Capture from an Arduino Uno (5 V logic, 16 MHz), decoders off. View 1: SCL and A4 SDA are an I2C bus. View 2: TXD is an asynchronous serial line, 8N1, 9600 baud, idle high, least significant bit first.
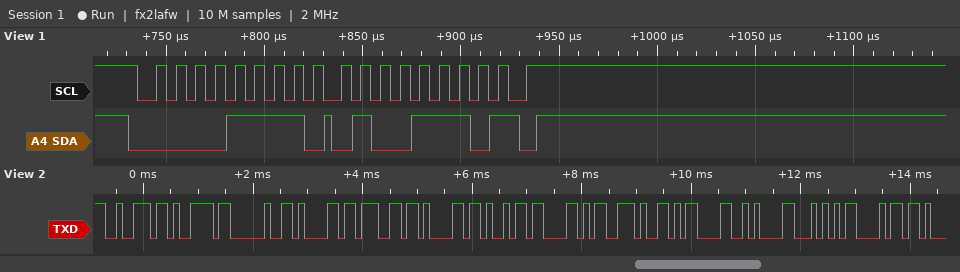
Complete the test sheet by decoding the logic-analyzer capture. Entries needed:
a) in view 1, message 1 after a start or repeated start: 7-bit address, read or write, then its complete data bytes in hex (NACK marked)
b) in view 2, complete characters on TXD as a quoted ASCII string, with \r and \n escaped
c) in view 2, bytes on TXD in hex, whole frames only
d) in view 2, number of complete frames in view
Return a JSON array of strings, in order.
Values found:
["0x07 read: 4E NACK", "\"ry agaiX.\\r\\nTh\"", "72 79 20 61 67 61 69 58 2E 0D 0A 54 68", "13"]
